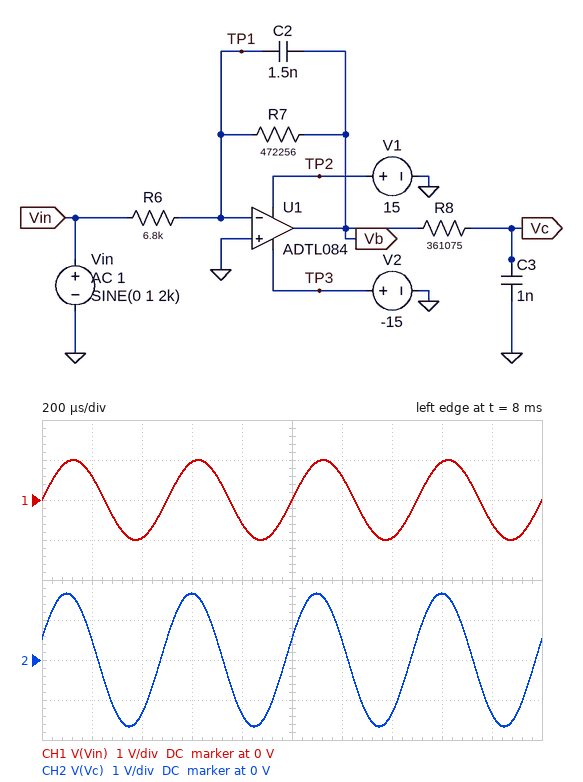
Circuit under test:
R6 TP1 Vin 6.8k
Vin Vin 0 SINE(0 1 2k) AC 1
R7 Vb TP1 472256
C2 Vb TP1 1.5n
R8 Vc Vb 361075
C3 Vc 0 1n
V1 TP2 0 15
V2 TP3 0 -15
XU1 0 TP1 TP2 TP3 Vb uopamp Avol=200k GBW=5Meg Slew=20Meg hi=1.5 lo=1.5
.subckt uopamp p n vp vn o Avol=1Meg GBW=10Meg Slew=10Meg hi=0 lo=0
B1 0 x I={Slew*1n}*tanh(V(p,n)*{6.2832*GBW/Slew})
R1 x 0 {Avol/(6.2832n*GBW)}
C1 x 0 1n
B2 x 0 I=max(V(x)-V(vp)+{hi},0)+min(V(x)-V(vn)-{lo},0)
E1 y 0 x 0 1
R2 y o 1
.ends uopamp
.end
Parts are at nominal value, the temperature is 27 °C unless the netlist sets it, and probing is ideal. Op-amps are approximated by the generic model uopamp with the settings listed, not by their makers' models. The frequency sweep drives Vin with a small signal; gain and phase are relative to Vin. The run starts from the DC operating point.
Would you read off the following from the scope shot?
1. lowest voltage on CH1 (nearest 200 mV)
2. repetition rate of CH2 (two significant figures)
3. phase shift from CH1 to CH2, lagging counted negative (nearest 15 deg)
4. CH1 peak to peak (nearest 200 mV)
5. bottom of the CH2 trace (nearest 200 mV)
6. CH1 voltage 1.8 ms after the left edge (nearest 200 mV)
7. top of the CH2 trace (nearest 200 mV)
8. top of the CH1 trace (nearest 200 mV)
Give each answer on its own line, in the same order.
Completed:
-1.0 V
2.0 kHz
15 deg
2.0 V
-1.6 V
-600 mV
1.6 V
1.0 V
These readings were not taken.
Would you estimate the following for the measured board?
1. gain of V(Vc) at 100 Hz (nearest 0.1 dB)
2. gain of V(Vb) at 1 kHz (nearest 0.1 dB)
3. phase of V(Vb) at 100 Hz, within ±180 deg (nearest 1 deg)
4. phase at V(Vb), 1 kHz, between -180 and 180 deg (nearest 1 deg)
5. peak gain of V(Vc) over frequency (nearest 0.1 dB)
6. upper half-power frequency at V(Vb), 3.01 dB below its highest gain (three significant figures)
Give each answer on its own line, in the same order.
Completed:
35.8 dB
23.6 dB
156 deg
103 deg
36.8 dB
224 Hz
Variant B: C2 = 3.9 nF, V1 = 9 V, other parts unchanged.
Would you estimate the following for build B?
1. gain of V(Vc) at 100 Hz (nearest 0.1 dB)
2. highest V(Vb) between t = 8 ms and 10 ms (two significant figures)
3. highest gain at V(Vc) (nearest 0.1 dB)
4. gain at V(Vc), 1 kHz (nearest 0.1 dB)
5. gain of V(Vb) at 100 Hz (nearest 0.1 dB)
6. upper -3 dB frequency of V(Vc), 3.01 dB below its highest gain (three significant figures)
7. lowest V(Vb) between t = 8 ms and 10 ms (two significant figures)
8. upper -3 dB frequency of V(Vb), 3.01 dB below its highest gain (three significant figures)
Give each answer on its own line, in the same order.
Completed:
32.9 dB
3.0 V
36.8 dB
7.6 dB
33.1 dB
83.3 Hz
-3.0 V
86.3 Hz
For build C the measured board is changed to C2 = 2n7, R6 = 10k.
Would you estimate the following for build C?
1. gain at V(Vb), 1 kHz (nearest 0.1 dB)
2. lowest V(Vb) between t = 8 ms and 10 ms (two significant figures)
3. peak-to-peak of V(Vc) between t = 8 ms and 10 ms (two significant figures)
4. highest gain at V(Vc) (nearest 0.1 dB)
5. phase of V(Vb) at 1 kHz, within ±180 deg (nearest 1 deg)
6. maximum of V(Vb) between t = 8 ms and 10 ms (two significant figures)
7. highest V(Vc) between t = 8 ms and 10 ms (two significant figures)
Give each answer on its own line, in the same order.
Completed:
15.3 dB
-2.9 V
1.3 V
33.5 dB
97 deg
2.9 V
630 mV
